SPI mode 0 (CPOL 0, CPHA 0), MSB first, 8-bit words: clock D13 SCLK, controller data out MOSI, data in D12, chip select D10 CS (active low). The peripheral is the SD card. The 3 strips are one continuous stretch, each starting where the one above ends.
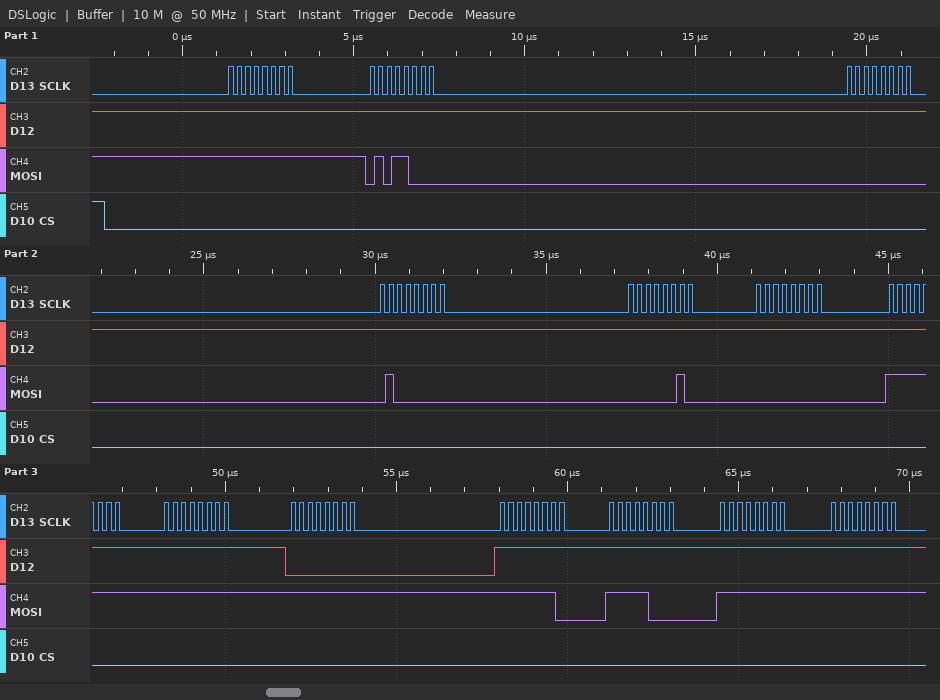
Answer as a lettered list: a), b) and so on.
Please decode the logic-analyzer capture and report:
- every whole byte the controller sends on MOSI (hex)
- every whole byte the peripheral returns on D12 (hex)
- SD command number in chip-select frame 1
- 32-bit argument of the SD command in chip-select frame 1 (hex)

a) 0xFF 0x58 0x00 0x40 0x02 0x00 0xFF 0xFF 0xFF 0xFE 0xF8 0xFF 0xFF
b) 0xFF 0xFF 0xFF 0xFF 0xFF 0xFF 0xFF 0xFF 0x00 0xFF 0xFF 0xFF 0xFF
c) CMD24
d) 0x00400200
